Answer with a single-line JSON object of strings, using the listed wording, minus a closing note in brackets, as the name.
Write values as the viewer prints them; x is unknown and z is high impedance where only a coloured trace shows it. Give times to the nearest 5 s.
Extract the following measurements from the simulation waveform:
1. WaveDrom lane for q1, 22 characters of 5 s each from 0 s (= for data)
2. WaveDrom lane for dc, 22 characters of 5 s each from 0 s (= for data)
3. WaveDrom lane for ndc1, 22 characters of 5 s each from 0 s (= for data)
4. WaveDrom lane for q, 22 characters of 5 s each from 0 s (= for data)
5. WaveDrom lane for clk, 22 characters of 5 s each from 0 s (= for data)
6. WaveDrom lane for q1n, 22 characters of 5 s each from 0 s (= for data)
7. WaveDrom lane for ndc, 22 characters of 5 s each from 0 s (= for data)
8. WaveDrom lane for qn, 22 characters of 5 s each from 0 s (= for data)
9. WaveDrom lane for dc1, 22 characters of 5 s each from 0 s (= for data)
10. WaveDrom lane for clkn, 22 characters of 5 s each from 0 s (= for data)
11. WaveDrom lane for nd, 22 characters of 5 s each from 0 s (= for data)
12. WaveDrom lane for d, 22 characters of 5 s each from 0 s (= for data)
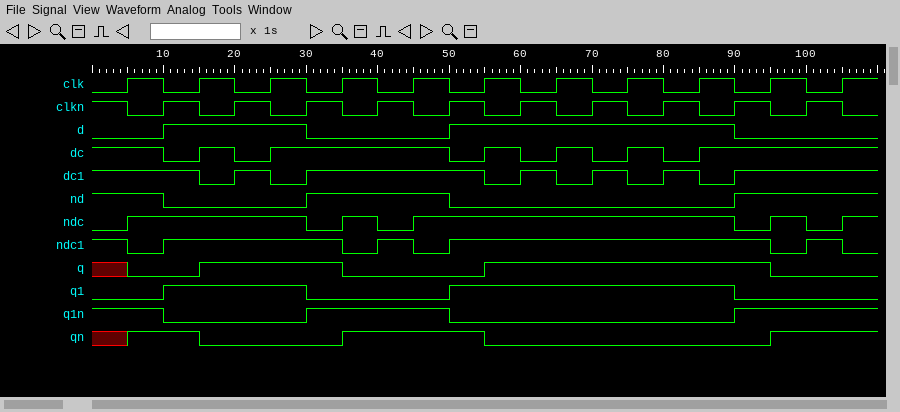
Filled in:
{"WaveDrom lane for q1, 22 characters of 5 s each from 0 s": "{name: 'q1', wave: '0.1...0...1.......0...'}", "WaveDrom lane for dc, 22 characters of 5 s each from 0 s": "{name: 'dc', wave: '1.0101....01010101....'}", "WaveDrom lane for ndc1, 22 characters of 5 s each from 0 s": "{name: 'ndc1', wave: '101....0101........010'}", "WaveDrom lane for q, 22 characters of 5 s each from 0 s": "{name: 'q', wave: 'x0.1...0...1.......0..'}", "WaveDrom lane for clk, 22 characters of 5 s each from 0 s": "{name: 'clk', wave: '0101010101010101010101'}", "WaveDrom lane for q1n, 22 characters of 5 s each from 0 s": "{name: 'q1n', wave: '1.0...1...0.......1...'}", "WaveDrom lane for ndc, 22 characters of 5 s each from 0 s": "{name: 'ndc', wave: '01....0101........0101'}", "WaveDrom lane for qn, 22 characters of 5 s each from 0 s": "{name: 'qn', wave: 'x1.0...1...0.......1..'}", "WaveDrom lane for dc1, 22 characters of 5 s each from 0 s": "{name: 'dc1', wave: '1..0101....01010101...'}", "WaveDrom lane for clkn, 22 characters of 5 s each from 0 s": "{name: 'clkn', wave: '1010101010101010101010'}", "WaveDrom lane for nd, 22 characters of 5 s each from 0 s": "{name: 'nd', wave: '1.0...1...0.......1...'}", "WaveDrom lane for d, 22 characters of 5 s each from 0 s": "{name: 'd', wave: '0.1...0...1.......0...'}"}
